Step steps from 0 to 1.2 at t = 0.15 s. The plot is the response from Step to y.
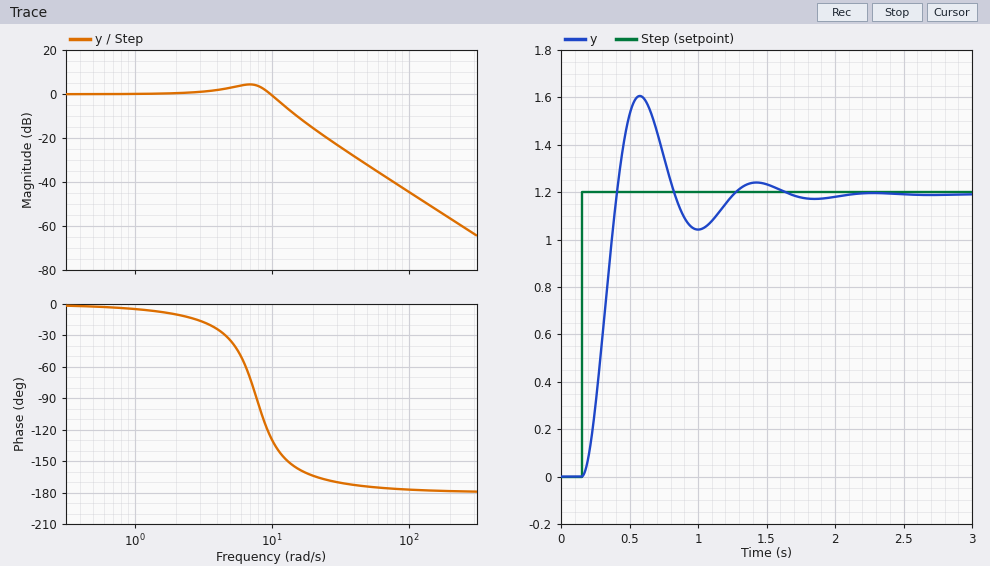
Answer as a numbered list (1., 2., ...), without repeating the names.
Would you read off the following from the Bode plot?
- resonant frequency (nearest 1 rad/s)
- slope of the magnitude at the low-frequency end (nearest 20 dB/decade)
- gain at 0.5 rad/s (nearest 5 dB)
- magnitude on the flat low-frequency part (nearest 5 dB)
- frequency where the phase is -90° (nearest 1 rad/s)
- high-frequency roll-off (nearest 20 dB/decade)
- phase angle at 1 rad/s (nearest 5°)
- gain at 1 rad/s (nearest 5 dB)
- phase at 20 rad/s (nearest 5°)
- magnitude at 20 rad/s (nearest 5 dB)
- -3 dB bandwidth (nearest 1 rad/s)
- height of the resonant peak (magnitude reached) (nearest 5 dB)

1. 7 rad/s
2. 0 dB/decade
3. 0 dB
4. 0 dB
5. 8 rad/s
6. -40 dB/decade
7. -5°
8. 0 dB
9. -165°
10. -15 dB
11. 11 rad/s
12. 5 dB
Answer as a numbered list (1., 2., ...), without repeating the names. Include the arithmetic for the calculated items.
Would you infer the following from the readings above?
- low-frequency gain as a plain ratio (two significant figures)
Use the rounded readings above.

1. 10^(0 / 20) = 1.0
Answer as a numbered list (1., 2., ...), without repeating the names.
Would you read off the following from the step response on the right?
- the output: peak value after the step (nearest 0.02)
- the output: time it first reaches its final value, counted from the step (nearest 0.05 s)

1. 1.60
2. 0.25 s
